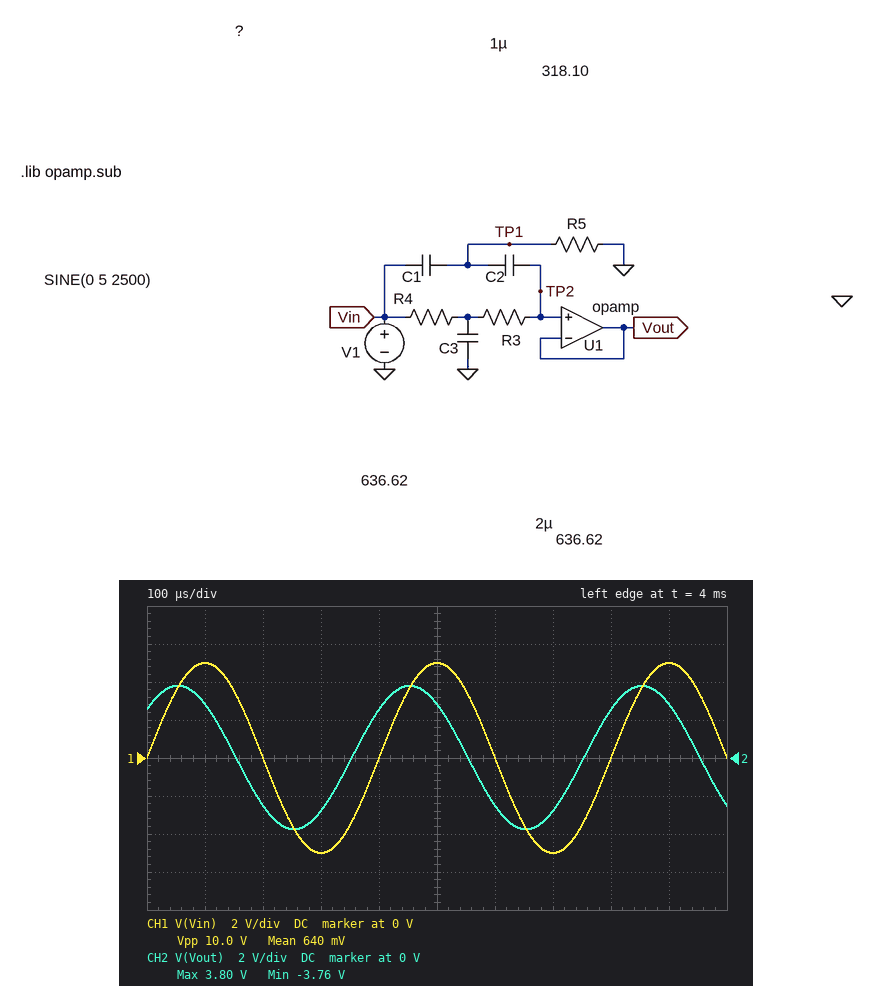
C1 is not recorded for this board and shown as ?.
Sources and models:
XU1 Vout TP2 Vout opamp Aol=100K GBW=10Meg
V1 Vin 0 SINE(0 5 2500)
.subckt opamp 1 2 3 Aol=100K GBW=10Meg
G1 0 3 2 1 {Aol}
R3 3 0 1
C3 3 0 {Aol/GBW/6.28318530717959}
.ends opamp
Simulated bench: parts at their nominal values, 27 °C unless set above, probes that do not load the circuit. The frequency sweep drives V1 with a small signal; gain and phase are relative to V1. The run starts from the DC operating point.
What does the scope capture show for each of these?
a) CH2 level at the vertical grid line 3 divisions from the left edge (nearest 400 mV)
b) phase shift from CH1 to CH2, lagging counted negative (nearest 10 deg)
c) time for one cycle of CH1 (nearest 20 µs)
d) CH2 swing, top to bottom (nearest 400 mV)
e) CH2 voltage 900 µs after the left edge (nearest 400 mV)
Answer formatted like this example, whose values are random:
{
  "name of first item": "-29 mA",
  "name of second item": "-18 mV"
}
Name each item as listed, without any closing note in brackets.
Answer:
{
  "CH2 level at the vertical grid line 3 divisions from the left edge": "-2.8 V",
  "phase shift from CH1 to CH2, lagging counted negative": "40 deg",
  "time for one cycle of CH1": "400 µs",
  "CH2 swing, top to bottom": "7.6 V",
  "CH2 voltage 900 µs after the left edge": "2.8 V"
}
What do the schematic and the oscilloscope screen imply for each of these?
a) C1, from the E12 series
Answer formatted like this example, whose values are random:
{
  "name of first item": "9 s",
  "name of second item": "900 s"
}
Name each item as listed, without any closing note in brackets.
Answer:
{
  "C1, from the E12 series": "390 nF"
}
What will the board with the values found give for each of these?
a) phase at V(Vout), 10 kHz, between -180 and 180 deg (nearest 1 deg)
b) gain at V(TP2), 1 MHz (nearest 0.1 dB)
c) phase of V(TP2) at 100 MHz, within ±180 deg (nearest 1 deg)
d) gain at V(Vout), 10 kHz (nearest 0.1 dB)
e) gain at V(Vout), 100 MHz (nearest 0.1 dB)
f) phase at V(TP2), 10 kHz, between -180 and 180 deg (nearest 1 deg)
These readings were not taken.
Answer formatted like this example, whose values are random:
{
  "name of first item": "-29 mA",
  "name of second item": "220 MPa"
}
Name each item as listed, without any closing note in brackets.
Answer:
{
  "phase at V(Vout), 10 kHz, between -180 and 180 deg": "12 deg",
  "gain at V(TP2), 1 MHz": "0 dB",
  "phase of V(TP2) at 100 MHz, within ±180 deg": "0 deg",
  "gain at V(Vout), 10 kHz": "-0.2 dB",
  "gain at V(Vout), 100 MHz": "-20.0 dB",
  "phase at V(TP2), 10 kHz, between -180 and 180 deg": "12 deg"
}
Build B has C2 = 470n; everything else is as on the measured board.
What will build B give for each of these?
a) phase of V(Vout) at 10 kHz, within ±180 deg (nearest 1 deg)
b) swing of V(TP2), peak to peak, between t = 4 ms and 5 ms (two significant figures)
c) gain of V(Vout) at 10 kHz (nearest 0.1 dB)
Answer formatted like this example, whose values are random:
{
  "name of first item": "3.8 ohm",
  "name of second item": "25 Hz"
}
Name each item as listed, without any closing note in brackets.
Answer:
{
  "phase of V(Vout) at 10 kHz, within ±180 deg": "14 deg",
  "swing of V(TP2), peak to peak, between t = 4 ms and 5 ms": "7.3 V",
  "gain of V(Vout) at 10 kHz": "-0.2 dB"
}
